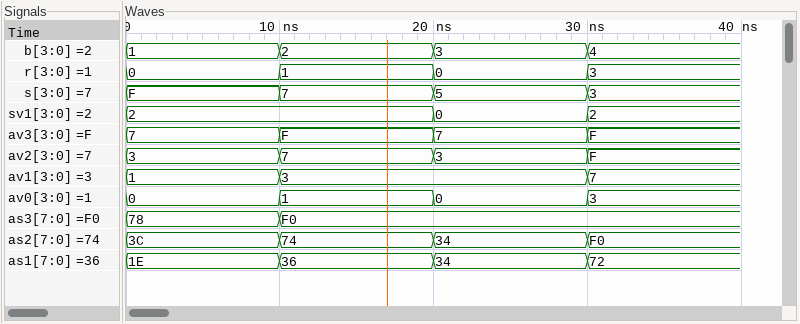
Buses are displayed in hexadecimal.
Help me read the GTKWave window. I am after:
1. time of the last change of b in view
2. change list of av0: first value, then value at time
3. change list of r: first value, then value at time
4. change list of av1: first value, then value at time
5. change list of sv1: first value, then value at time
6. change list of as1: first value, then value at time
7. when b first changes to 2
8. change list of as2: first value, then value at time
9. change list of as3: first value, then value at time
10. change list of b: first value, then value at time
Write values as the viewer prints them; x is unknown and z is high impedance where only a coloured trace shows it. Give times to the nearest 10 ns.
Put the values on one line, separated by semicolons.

30 ns; 0, 1 at 10 ns, 0 at 20 ns, 3 at 30 ns; 0, 1 at 10 ns, 0 at 20 ns, 3 at 30 ns; 1, 3 at 10 ns, 7 at 30 ns; 2, 0 at 20 ns, 2 at 30 ns; 1E, 36 at 10 ns, 34 at 20 ns, 72 at 30 ns; 10 ns; 3C, 74 at 10 ns, 34 at 20 ns, F0 at 30 ns; 78, F0 at 10 ns; 1, 2 at 10 ns, 3 at 20 ns, 4 at 30 ns
